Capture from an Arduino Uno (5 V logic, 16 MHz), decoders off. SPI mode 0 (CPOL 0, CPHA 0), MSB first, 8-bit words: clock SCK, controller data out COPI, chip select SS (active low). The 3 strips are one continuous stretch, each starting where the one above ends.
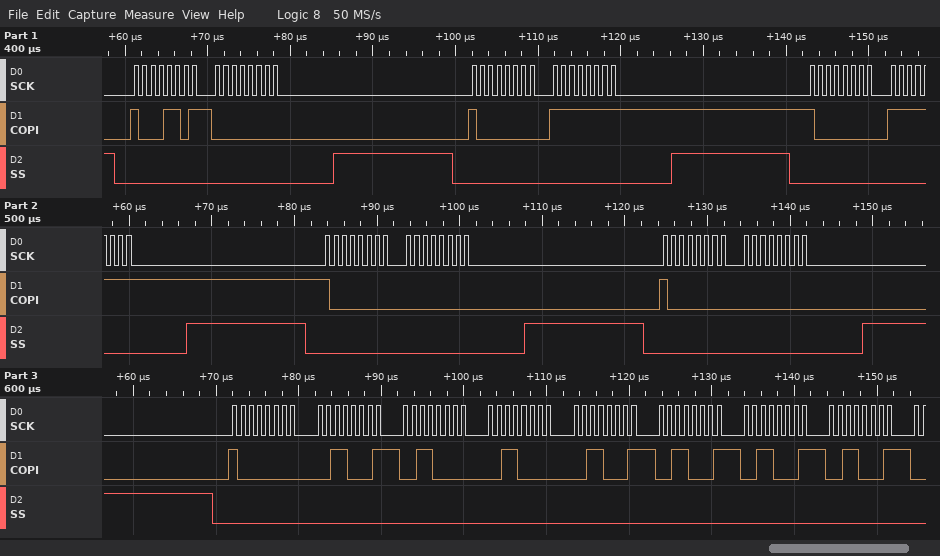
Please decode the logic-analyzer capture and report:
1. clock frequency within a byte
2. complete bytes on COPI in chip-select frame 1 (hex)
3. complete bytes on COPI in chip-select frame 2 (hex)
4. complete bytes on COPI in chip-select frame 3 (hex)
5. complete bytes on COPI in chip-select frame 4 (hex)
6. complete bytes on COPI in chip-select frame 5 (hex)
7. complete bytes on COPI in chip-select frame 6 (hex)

1 MHz
0x8D 0x00
0x80 0xFF
0x80 0xFF
0x80 0x00
0x80 0x00
0x80 0x31 0x30 0x30 0x31 0x31 0x31 0x31
